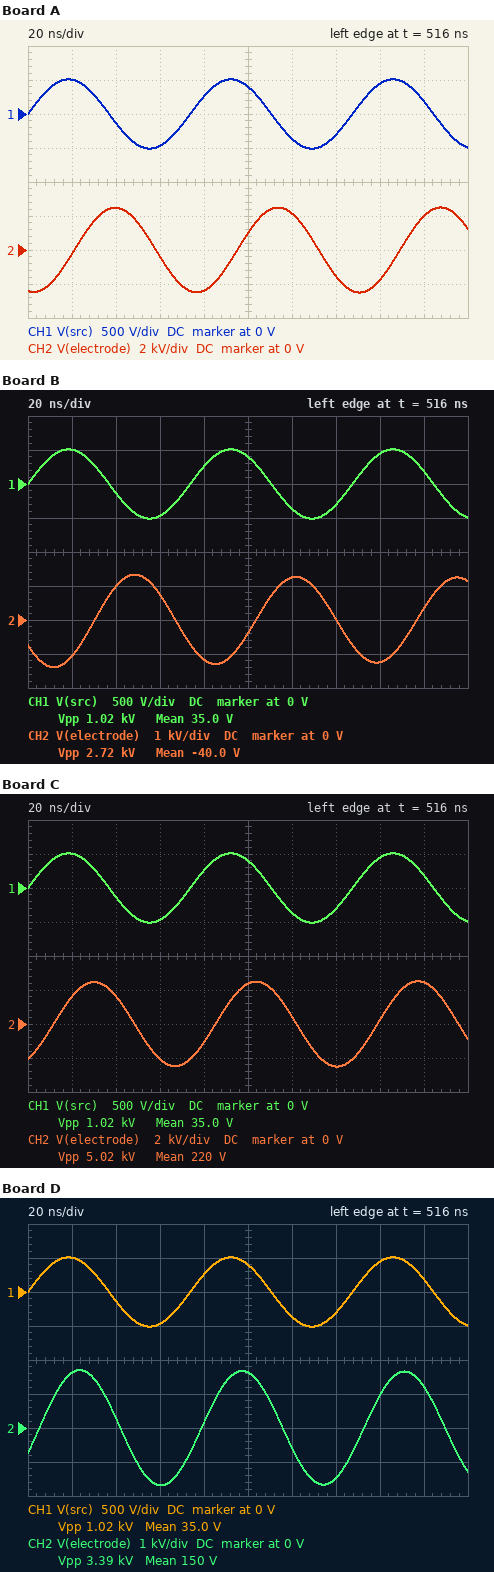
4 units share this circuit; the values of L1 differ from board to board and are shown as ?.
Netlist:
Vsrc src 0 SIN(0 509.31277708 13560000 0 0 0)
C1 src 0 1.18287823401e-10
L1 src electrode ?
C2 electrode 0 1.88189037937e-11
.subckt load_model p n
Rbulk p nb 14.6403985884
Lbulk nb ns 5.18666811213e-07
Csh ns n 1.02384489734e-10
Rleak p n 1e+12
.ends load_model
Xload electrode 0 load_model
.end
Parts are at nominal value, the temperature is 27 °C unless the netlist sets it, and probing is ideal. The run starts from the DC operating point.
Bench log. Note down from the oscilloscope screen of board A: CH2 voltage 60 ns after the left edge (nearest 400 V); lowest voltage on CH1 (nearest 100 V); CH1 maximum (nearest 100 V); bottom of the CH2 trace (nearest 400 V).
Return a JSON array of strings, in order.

["-400 V", "-500 V", "500 V", "-2.4 kV"]
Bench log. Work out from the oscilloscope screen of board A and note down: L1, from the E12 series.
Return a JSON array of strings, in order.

["820 nH"]
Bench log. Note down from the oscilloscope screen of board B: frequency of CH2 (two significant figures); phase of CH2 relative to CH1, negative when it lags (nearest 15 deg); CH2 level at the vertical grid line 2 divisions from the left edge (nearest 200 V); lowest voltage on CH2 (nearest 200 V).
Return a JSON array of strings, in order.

["14 MHz", "-150 deg", "1.0 kV", "-1.4 kV"]
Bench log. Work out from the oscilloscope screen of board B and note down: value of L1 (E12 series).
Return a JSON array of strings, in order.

["1 µH"]
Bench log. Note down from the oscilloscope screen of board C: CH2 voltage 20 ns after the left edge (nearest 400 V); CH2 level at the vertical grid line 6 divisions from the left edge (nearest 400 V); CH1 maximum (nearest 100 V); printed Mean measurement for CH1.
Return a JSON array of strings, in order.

["1.6 kV", "400 V", "500 V", "35.0 V"]
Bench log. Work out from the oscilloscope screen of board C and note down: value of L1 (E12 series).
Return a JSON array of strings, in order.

["680 nH"]
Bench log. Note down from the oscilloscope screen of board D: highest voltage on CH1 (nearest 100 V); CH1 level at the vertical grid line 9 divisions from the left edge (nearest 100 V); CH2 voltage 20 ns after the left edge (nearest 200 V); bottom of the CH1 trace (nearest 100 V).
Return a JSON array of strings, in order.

["500 V", "200 V", "1.6 kV", "-500 V"]
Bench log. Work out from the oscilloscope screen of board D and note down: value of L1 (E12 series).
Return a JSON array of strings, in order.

["560 nH"]
